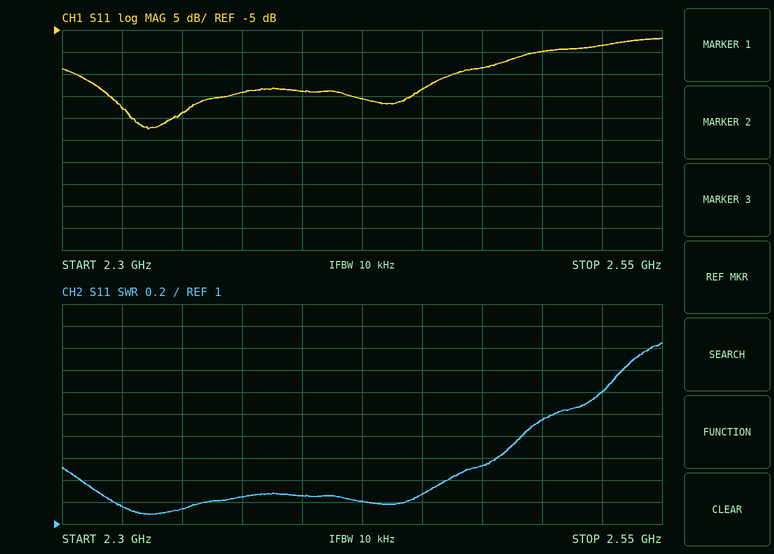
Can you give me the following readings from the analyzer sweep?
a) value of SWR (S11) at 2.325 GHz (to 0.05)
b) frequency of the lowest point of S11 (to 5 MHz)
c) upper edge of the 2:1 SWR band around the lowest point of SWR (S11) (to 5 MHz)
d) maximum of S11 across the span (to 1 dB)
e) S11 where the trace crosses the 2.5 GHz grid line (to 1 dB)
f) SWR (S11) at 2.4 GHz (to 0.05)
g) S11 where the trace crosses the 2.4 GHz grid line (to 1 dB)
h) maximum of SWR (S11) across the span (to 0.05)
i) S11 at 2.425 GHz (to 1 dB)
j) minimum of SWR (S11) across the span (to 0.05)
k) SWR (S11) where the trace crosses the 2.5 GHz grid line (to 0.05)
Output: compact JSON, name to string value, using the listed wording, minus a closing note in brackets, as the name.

{"value of SWR (S11) at 2.325 GHz": "1.15", "frequency of the lowest point of S11": "2.335 GHz", "upper edge of the 2:1 SWR band around the lowest point of SWR (S11)": "2.505 GHz", "maximum of S11 across the span": "-7 dB", "S11 where the trace crosses the 2.5 GHz grid line": "-10 dB", "SWR (S11) at 2.4 GHz": "1.25", "S11 where the trace crosses the 2.4 GHz grid line": "-19 dB", "maximum of SWR (S11) across the span": "2.65", "S11 at 2.425 GHz": "-21 dB", "minimum of SWR (S11) across the span": "1.10", "SWR (S11) where the trace crosses the 2.5 GHz grid line": "1.95"}
